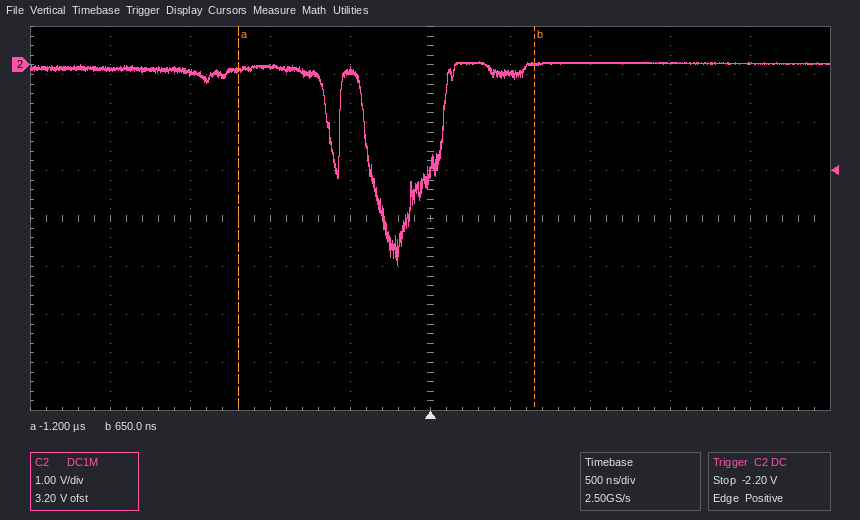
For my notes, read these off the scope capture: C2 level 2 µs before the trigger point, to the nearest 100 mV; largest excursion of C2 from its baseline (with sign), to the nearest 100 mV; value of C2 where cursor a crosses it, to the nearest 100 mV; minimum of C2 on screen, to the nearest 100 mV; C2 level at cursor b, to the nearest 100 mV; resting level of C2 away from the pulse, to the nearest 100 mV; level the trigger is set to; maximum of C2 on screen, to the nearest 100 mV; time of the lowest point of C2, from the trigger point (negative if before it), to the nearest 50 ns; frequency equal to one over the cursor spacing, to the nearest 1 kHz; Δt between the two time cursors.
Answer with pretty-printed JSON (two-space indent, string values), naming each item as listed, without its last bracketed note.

{
  "C2 level 2 µs before the trigger point, to the nearest 100 mV": "-100 mV",
  "largest excursion of C2 from its baseline (with sign), to the nearest 100 mV": "-4.2 V",
  "value of C2 where cursor a crosses it, to the nearest 100 mV": "-100 mV",
  "minimum of C2 on screen, to the nearest 100 mV": "-4.2 V",
  "C2 level at cursor b, to the nearest 100 mV": "0.0 V",
  "resting level of C2 away from the pulse, to the nearest 100 mV": "0.0 V",
  "level the trigger is set to": "-2.20 V",
  "maximum of C2 on screen, to the nearest 100 mV": "100 mV",
  "time of the lowest point of C2, from the trigger point (negative if before it), to the nearest 50 ns": "-200 ns",
  "frequency equal to one over the cursor spacing, to the nearest 1 kHz": "541 kHz",
  "Δt between the two time cursors": "1.85 µs"
}
